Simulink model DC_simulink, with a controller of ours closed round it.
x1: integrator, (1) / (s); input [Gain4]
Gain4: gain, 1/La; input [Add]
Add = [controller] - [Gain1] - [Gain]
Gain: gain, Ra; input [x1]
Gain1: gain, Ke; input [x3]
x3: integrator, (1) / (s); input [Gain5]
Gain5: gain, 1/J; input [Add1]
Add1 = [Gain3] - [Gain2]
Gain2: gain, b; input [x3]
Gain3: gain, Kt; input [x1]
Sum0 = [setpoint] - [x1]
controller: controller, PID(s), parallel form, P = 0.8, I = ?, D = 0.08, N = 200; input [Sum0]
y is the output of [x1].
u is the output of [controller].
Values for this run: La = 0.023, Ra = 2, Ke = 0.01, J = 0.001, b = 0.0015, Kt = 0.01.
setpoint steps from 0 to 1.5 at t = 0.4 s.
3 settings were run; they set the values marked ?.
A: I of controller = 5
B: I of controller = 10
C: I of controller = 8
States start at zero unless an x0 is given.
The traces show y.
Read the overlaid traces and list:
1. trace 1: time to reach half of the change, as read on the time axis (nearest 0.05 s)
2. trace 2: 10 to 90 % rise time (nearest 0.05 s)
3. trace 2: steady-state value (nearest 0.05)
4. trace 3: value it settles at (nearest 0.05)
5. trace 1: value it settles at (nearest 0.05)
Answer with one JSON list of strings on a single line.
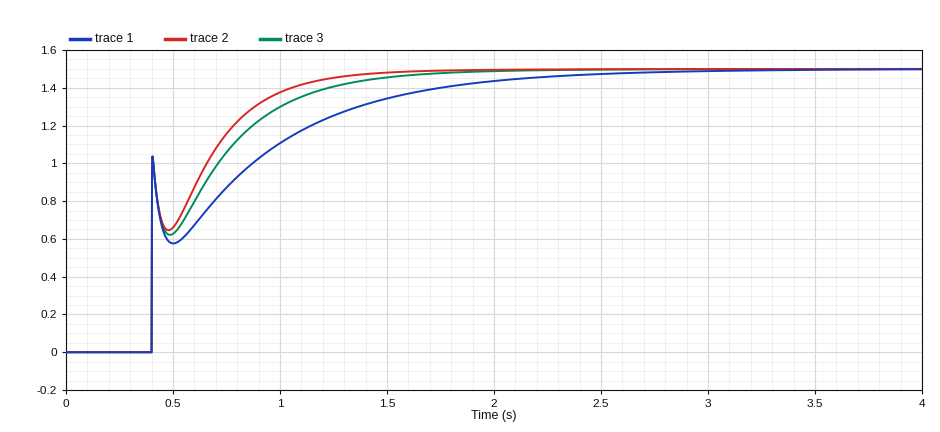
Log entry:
["0.40 s", "0.55 s", "1.50", "1.50", "1.50"]
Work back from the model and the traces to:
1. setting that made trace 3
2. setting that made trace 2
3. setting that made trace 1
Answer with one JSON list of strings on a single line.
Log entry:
["C", "B", "A"]
